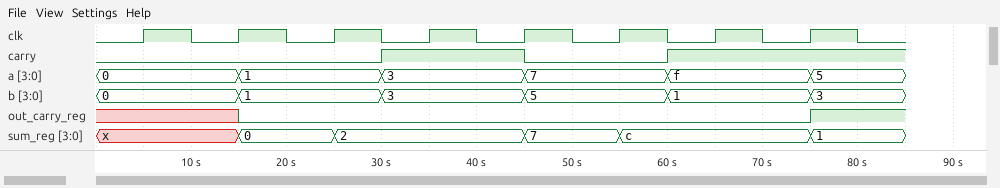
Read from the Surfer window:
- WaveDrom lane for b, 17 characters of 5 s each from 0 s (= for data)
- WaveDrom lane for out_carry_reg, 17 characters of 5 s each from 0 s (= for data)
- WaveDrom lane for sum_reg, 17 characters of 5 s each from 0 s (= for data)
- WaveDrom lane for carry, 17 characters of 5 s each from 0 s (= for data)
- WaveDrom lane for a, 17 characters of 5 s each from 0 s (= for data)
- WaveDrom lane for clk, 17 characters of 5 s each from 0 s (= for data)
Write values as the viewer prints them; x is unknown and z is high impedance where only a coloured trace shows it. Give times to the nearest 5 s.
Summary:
{name: 'b', wave: '=..=..=..=..=..=.', data: '0 1 3 5 1 3'}
{name: 'out_carry_reg', wave: 'x..0...........1.'}
{name: 'sum_reg', wave: 'x..=.=...=.=...=.', data: '0 2 7 c 1'}
{name: 'carry', wave: '0.....1..0..1....'}
{name: 'a', wave: '=..=..=..=..=..=.', data: '0 1 3 7 f 5'}
{name: 'clk', wave: '01010101010101010'}
